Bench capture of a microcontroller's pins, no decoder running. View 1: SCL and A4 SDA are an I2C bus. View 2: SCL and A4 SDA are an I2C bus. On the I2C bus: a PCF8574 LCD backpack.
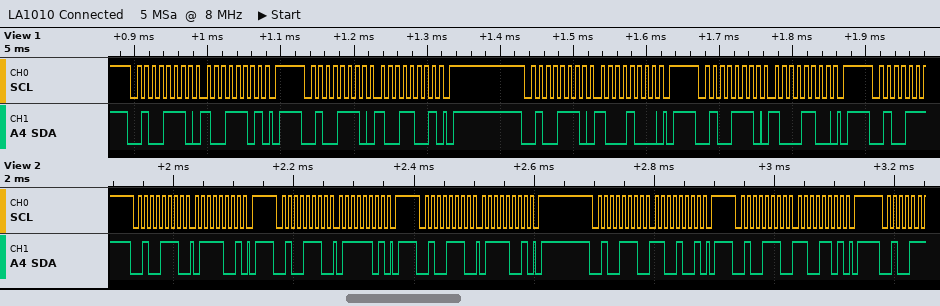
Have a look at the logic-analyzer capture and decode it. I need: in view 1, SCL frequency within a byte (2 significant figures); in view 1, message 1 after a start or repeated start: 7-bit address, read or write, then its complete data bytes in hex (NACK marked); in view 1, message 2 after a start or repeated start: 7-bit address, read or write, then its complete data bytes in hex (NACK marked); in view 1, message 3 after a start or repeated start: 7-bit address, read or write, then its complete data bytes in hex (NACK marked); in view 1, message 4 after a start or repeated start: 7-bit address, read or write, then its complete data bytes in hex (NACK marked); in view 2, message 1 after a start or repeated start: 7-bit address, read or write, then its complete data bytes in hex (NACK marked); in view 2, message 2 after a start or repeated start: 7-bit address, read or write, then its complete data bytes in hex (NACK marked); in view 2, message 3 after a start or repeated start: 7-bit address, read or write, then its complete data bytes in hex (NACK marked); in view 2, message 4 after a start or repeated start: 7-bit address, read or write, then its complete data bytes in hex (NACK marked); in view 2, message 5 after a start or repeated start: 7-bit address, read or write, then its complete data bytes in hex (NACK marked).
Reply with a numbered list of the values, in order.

1. 100 kHz
2. 0x27 write: 9D
3. 0x27 write: 99
4. 0x27 write: 88
5. 0x27 write: 8C
6. 0x27 write: 79
7. 0x27 write: 7D
8. 0x27 write: 79
9. 0x27 write: C9
10. 0x27 write: CD
